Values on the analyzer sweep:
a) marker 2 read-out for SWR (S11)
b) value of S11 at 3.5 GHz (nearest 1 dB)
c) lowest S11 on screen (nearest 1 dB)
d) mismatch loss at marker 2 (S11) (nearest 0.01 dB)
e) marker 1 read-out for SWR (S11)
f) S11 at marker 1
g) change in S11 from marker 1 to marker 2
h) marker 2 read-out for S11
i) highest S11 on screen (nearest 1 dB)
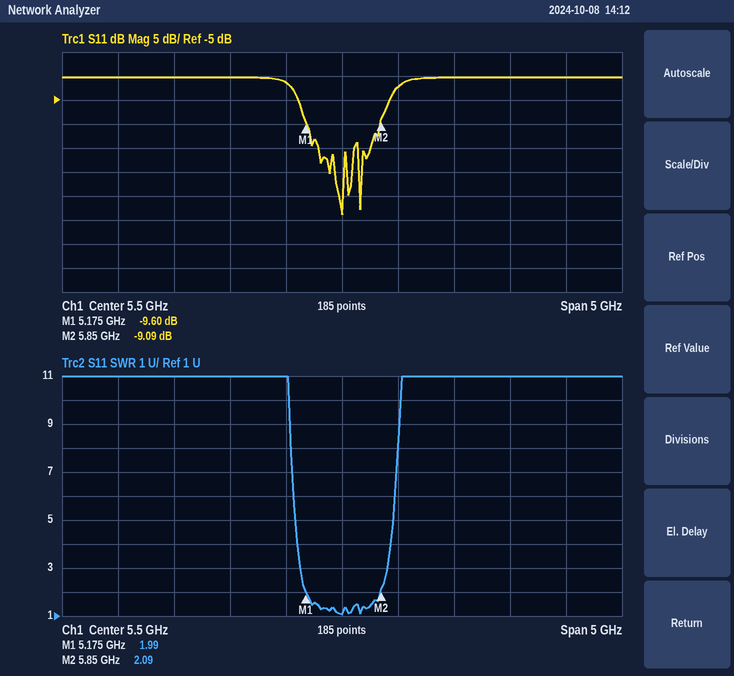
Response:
2.09
0 dB
-29 dB
0.57 dB
1.99
-9.60 dB
0.51 dB
-9.09 dB
0 dB
